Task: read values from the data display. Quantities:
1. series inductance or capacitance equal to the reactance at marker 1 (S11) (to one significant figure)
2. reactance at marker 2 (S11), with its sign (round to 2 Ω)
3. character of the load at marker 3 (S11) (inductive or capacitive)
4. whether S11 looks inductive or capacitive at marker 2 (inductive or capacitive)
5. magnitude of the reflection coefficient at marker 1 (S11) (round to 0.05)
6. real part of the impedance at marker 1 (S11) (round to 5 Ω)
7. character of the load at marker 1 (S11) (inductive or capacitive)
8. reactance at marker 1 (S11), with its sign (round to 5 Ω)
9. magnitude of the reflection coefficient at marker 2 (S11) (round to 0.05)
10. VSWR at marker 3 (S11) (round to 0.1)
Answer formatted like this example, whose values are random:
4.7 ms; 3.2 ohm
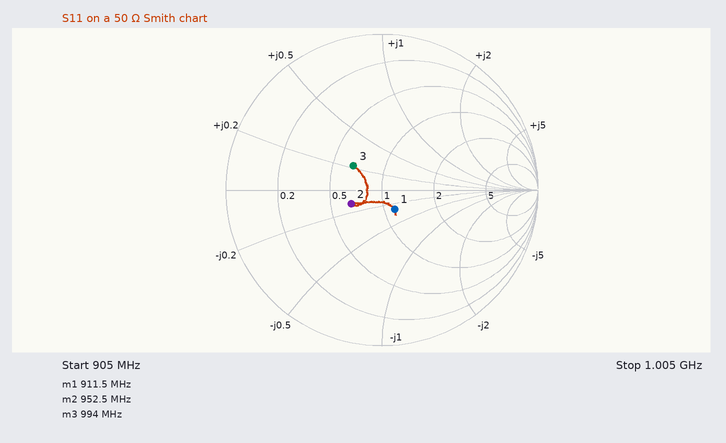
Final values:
10 pF; -6 Ω; inductive; capacitive; 0.15; 55 Ω; capacitive; -15 Ω; 0.20; 1.6
